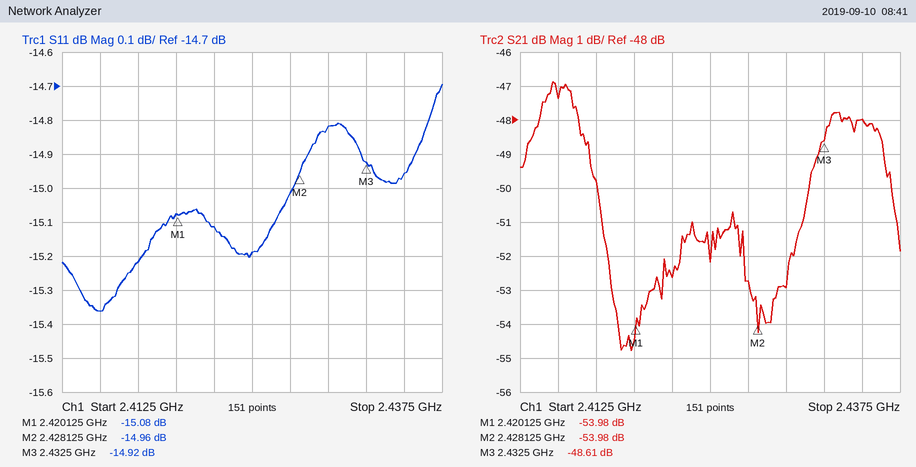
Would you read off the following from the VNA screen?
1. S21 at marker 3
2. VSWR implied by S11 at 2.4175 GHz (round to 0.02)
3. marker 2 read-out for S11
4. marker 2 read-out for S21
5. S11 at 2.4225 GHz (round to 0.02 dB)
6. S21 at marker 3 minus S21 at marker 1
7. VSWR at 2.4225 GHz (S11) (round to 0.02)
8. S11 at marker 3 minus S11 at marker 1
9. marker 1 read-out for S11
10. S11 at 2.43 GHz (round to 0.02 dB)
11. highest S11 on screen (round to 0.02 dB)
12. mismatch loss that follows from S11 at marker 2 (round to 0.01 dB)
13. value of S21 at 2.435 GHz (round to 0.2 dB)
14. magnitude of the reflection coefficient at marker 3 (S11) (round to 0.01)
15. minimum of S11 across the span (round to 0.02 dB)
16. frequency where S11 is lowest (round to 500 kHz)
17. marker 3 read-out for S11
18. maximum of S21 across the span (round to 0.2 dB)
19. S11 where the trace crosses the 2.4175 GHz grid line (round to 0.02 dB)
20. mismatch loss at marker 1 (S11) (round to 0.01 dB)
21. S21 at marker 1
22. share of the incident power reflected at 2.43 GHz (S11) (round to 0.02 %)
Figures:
-48.61 dB
1.42
-14.96 dB
-53.98 dB
-15.12 dB
5.37 dB
1.42
0.16 dB
-15.08 dB
-14.82 dB
-14.70 dB
0.14 dB
-48.0 dB
0.18
-15.36 dB
2.4150 GHz
-14.92 dB
-46.8 dB
-15.22 dB
0.14 dB
-53.98 dB
3.30 %
